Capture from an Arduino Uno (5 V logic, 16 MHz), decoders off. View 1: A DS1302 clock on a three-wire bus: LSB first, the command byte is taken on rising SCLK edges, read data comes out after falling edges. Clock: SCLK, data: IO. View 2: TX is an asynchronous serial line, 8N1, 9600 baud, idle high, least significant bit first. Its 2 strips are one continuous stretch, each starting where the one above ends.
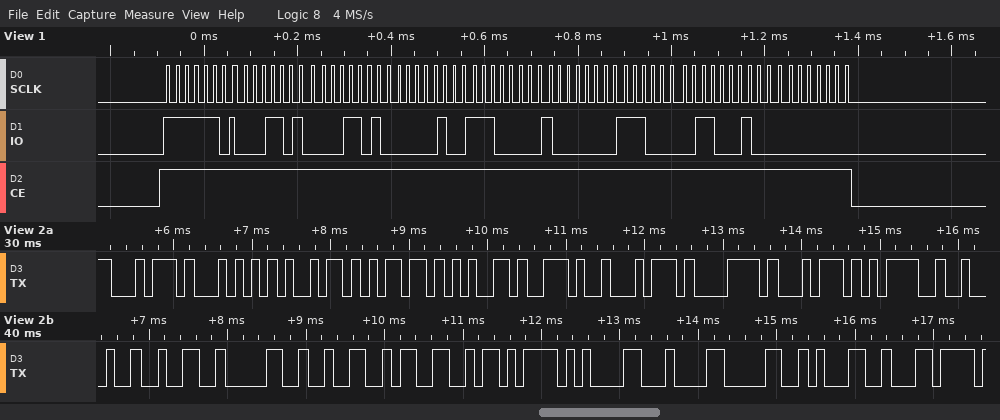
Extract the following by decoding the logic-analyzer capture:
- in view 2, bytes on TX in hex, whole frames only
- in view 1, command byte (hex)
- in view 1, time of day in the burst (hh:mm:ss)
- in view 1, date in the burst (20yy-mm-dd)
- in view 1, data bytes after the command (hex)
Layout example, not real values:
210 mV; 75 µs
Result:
0x74 0x54 0x69 0x6D 0x65 0x2E 0x74 0x78 0x74 0x3D 0x22 0x32 0x30 0x32 0x33 0xEB 0x85 0x84 0x30 0x31 0xEC; 0xBF; 20:58:58; 2023-01-07; 58 58 20 07 01 07 23 00
